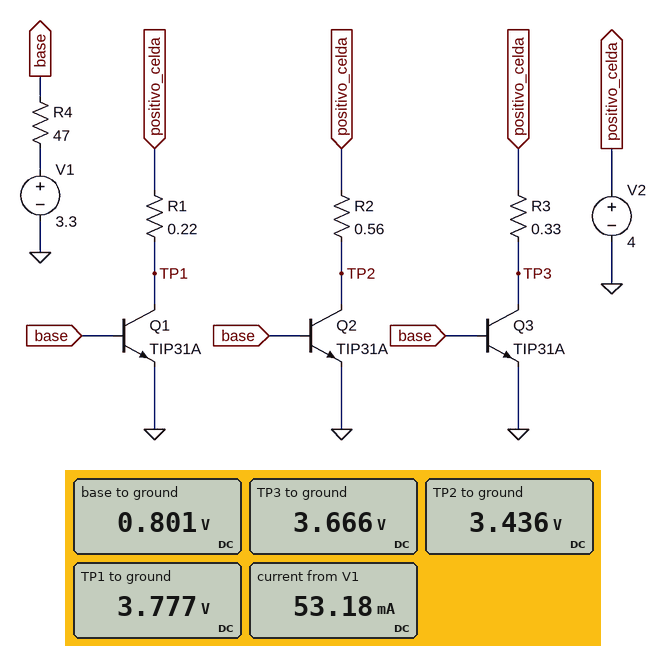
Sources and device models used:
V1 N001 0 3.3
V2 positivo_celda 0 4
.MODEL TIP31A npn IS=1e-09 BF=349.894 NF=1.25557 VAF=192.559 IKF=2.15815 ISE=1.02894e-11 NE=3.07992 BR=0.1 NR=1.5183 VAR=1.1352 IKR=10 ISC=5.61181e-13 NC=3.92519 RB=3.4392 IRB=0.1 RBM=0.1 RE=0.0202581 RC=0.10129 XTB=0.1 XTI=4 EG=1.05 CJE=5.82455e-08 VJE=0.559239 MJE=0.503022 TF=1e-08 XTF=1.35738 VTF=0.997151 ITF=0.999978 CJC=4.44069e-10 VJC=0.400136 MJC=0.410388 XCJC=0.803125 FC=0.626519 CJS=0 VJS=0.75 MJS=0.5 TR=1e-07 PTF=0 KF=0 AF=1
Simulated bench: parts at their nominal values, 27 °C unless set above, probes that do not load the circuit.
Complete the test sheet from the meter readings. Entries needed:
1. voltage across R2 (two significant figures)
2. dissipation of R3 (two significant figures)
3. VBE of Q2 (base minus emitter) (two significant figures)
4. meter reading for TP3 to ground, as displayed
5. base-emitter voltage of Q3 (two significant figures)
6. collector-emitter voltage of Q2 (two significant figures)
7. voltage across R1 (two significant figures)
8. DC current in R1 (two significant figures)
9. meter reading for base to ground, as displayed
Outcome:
560 mV
340 mW
800 mV
3.666 V
800 mV
3.4 V
220 mV
1.0 A
0.801 V
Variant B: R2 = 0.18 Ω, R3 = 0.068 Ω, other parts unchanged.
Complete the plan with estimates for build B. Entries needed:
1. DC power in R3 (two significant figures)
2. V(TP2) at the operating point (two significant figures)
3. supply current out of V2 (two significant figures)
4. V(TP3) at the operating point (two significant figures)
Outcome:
70 mW
3.8 V
3.0 A
3.9 V
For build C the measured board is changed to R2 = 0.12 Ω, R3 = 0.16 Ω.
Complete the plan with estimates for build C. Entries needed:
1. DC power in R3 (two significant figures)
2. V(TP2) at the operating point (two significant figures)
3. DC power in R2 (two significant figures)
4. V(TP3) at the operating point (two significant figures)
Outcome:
160 mW
3.9 V
120 mW
3.8 V
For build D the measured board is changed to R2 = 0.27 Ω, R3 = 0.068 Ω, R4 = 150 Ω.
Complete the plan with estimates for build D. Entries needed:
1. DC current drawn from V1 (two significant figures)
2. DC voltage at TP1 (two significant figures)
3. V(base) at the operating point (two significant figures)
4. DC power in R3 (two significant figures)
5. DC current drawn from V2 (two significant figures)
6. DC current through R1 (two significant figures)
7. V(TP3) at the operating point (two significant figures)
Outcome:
17 mA
3.9 V
720 mV
18 mW
1.5 A
510 mA
4.0 V
